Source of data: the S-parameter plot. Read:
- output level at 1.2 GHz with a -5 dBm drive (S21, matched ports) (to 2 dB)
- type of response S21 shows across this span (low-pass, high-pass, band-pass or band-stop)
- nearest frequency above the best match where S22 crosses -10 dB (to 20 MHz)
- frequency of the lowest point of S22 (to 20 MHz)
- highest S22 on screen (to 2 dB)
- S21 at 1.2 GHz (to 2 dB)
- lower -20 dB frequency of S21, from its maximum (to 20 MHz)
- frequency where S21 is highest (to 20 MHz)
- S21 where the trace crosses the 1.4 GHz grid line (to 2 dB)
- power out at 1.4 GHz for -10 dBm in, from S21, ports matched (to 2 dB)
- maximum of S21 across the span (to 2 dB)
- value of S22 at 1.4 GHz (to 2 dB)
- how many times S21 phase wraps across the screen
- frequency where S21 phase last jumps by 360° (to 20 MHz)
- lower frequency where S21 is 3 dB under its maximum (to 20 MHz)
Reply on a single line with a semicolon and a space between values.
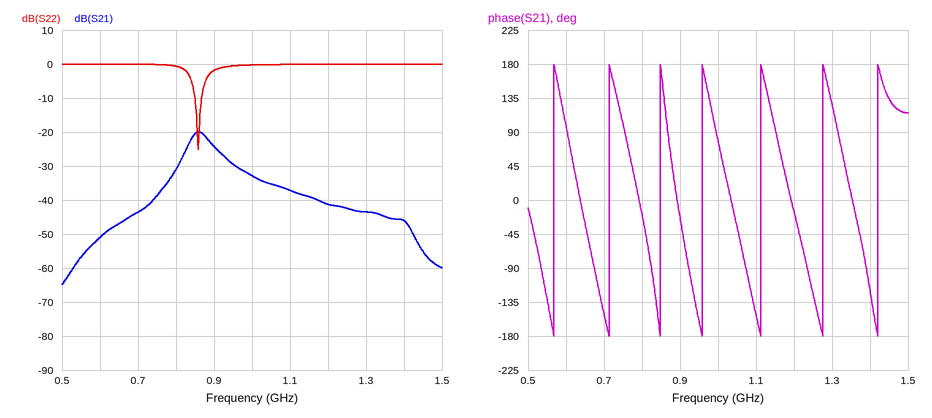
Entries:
-46 dBm; band-pass; 860 MHz; 860 MHz; 0 dB; -42 dB; 740 MHz; 860 MHz; -46 dB; -56 dBm; -20 dB; 0 dB; 7; 1.42 GHz; 840 MHz
